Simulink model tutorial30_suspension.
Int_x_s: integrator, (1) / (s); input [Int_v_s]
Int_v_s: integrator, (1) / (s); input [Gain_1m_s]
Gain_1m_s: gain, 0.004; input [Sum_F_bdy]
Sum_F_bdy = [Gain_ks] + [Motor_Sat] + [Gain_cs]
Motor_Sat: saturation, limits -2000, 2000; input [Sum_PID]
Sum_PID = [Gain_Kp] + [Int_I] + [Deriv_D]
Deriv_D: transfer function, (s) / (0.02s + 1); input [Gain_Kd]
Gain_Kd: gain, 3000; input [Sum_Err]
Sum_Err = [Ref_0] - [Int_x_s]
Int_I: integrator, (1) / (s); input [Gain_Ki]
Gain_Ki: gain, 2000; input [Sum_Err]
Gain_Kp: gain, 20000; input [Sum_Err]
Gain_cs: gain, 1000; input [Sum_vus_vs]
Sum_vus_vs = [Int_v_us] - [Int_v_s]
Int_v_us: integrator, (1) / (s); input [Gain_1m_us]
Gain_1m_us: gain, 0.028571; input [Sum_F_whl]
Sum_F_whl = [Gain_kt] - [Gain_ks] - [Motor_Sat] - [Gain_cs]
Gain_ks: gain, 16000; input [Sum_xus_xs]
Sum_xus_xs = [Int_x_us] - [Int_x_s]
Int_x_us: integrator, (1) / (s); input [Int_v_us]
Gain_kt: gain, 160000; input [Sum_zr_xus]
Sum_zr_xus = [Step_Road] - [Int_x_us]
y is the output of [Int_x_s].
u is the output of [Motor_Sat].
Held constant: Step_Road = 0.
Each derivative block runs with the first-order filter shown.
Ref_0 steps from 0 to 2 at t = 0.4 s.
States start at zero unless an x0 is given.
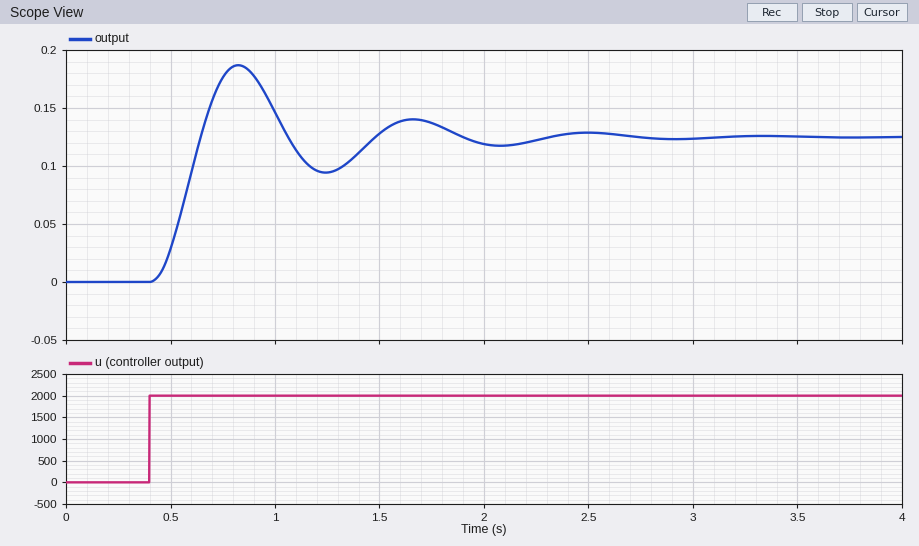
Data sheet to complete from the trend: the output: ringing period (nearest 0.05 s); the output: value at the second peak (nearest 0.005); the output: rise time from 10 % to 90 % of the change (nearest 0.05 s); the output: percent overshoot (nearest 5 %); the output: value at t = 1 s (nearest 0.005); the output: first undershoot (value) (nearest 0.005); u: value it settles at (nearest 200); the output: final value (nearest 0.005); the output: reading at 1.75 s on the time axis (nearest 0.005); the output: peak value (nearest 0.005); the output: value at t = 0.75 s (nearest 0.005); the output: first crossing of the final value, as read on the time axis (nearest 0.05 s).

0.85 s
0.140
0.15 s
50 %
0.145
0.095
2000
0.125
0.135
0.185
0.175
0.65 s
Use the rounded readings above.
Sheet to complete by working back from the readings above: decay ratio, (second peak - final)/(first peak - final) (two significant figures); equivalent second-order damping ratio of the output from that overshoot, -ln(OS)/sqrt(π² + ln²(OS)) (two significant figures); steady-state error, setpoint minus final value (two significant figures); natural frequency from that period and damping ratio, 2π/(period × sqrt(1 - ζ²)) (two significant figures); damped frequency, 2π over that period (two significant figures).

0.25
0.22
1.9
7.6 rad/s
7.4 rad/s
